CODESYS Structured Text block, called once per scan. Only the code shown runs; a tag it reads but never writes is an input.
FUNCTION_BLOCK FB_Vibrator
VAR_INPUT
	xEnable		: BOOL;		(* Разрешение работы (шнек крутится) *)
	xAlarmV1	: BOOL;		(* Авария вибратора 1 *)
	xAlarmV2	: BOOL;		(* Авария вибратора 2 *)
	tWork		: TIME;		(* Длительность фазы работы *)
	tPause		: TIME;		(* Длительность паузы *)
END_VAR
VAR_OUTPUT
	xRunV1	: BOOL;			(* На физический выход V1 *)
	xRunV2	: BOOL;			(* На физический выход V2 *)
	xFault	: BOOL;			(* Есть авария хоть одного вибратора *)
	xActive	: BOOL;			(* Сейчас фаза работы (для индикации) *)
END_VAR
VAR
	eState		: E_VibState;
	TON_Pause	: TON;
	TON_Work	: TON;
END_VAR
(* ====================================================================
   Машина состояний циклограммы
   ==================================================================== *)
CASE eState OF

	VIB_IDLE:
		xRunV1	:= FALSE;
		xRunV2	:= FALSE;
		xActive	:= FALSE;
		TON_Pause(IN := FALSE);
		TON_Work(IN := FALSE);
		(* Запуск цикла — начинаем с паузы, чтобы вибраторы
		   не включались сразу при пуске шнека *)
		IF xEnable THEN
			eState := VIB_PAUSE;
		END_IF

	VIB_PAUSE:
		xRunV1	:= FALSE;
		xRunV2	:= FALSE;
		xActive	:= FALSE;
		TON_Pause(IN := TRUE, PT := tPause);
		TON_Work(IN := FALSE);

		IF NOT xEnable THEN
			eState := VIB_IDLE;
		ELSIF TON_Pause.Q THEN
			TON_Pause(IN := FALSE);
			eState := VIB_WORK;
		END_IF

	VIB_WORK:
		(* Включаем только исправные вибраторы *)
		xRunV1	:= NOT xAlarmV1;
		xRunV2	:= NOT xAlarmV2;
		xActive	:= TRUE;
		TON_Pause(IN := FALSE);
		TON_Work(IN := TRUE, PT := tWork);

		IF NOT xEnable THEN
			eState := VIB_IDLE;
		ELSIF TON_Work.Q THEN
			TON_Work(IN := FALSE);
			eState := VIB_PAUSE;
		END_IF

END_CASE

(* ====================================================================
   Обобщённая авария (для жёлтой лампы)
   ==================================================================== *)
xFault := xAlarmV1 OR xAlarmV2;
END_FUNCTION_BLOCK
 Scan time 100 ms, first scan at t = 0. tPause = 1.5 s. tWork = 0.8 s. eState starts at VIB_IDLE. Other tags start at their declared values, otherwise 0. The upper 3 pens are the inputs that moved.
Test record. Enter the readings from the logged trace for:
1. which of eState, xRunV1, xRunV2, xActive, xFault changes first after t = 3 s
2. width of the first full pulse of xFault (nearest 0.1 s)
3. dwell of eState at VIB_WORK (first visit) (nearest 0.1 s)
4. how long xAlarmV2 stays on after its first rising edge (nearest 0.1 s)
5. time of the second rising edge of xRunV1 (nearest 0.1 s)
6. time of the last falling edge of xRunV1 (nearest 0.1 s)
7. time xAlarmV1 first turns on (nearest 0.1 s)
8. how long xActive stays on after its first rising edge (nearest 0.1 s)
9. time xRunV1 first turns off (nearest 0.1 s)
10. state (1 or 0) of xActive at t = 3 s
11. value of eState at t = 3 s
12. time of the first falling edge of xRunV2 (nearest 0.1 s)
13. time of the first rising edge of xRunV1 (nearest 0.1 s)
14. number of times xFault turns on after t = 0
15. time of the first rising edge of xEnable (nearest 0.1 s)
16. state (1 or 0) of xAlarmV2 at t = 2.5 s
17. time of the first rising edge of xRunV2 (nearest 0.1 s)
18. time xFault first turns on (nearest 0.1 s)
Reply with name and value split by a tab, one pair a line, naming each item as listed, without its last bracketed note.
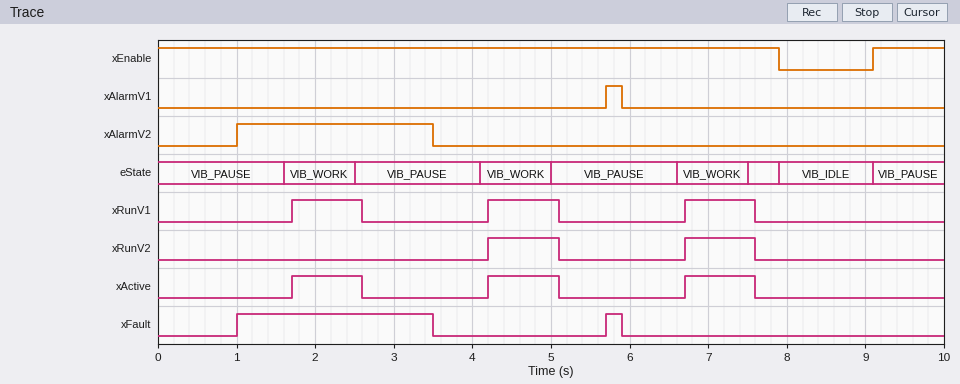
which of eState, xRunV1, xRunV2, xActive, xFault changes first after t = 3 s	xFault
width of the first full pulse of xFault	2.5 s
dwell of eState at VIB_WORK (first visit)	0.9 s
how long xAlarmV2 stays on after its first rising edge	2.5 s
time of the second rising edge of xRunV1	4.2 s
time of the last falling edge of xRunV1	7.6 s
time xAlarmV1 first turns on	5.7 s
how long xActive stays on after its first rising edge	0.9 s
time xRunV1 first turns off	2.6 s
state (1 or 0) of xActive at t = 3 s	0
value of eState at t = 3 s	VIB_PAUSE
time of the first falling edge of xRunV2	5.1 s
time of the first rising edge of xRunV1	1.7 s
number of times xFault turns on after t = 0	2
time of the first rising edge of xEnable	9.1 s
state (1 or 0) of xAlarmV2 at t = 2.5 s	1
time of the first rising edge of xRunV2	4.2 s
time xFault first turns on	1.0 s
